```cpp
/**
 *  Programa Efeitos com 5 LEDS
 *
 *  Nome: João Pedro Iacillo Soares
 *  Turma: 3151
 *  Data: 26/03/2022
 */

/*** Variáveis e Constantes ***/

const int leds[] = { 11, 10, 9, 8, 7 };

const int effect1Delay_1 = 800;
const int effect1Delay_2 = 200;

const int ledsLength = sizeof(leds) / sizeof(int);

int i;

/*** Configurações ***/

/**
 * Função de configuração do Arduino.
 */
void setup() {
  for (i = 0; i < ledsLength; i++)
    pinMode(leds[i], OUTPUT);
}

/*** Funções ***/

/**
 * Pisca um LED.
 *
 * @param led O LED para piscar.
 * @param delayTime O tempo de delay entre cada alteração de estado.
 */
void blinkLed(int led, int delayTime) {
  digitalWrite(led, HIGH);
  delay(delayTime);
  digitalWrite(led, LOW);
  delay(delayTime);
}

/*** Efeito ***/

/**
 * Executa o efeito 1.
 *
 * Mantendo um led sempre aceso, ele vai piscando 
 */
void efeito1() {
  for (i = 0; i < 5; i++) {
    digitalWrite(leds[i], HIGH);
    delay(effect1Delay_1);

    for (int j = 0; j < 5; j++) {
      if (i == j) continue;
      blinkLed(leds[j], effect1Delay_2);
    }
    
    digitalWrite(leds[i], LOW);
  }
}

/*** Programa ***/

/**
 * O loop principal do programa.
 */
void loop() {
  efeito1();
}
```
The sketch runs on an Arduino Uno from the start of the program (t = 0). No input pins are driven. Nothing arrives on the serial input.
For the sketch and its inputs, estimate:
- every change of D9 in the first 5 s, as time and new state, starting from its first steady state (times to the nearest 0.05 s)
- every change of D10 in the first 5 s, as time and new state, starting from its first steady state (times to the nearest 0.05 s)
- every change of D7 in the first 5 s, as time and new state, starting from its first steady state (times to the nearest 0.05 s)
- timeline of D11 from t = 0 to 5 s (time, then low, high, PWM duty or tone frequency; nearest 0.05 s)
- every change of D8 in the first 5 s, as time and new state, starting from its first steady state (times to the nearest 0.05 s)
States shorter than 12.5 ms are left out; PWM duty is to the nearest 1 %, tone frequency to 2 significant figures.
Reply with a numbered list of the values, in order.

1. 0 s low; 1.2 s high; 1.4 s low; 3.6 s high; 3.8 s low; 4.8 s high
2. 0 s low; 0.8 s high; 1 s low; 2.4 s high; 4.8 s low
3. 0 s low; 2 s high; 2.2 s low; 4.4 s high; 4.6 s low
4. 0 s high; 2.4 s low; 3.2 s high; 3.4 s low
5. 0 s low; 1.6 s high; 1.8 s low; 4 s high; 4.2 s low
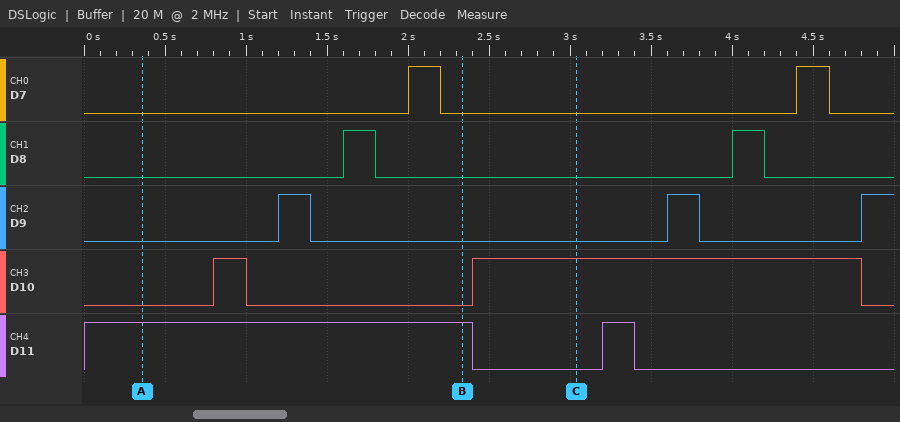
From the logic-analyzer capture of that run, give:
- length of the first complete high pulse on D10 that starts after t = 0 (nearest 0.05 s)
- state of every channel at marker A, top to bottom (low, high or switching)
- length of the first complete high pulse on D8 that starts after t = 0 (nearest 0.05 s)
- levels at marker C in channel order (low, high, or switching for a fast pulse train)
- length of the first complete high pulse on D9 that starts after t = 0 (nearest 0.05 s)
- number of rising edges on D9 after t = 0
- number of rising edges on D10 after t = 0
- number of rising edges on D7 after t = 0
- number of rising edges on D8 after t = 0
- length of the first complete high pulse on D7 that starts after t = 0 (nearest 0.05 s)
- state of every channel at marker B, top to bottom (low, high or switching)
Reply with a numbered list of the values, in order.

1. 0.20 s
2. D7 low, D8 low, D9 low, D10 low, D11 high
3. 0.20 s
4. D7 low, D8 low, D9 low, D10 high, D11 low
5. 0.20 s
6. 3
7. 2
8. 2
9. 2
10. 0.20 s
11. D7 low, D8 low, D9 low, D10 low, D11 high
